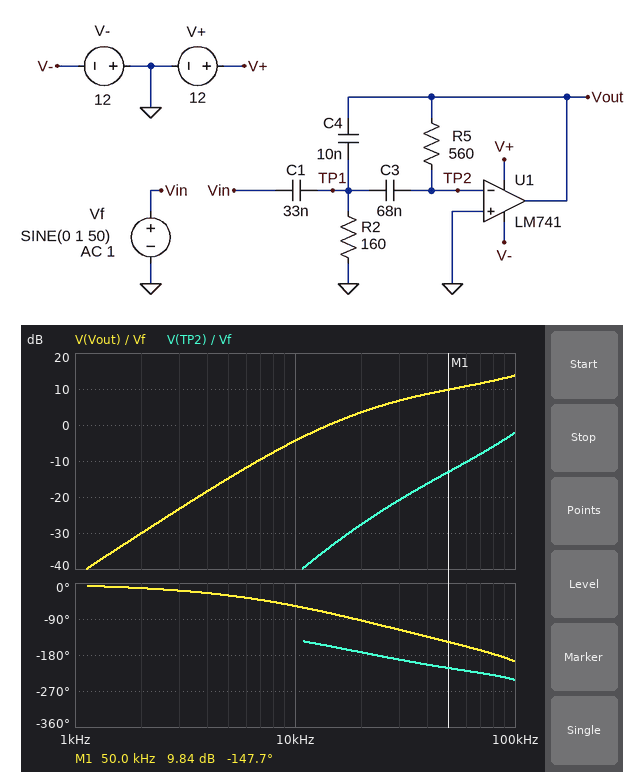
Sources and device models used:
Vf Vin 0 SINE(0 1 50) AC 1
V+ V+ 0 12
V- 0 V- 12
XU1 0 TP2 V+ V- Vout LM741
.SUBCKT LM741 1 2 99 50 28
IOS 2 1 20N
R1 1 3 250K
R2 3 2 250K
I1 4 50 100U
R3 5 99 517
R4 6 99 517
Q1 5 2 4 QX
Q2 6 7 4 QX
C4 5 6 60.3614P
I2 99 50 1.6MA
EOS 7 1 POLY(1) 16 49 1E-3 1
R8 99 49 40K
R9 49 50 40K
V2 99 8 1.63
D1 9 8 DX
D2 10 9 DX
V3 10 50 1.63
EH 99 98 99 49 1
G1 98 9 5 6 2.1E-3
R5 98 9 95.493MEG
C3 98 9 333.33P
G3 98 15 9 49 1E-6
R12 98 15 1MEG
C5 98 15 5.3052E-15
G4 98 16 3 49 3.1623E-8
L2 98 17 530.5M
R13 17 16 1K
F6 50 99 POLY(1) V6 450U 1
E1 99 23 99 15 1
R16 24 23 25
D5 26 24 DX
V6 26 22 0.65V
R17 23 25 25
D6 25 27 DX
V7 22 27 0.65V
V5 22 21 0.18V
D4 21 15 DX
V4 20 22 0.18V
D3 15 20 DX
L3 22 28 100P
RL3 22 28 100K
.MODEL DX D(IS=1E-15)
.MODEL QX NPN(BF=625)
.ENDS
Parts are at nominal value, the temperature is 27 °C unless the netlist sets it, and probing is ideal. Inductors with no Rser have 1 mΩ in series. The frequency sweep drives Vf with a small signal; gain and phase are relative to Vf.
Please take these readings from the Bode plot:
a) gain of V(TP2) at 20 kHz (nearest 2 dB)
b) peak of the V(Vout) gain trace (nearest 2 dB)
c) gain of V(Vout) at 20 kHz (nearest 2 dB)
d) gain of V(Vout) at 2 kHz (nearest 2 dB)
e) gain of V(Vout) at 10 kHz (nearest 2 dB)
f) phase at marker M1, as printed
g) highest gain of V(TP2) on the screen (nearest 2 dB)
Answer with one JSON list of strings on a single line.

["-28 dB", "14 dB", "4 dB", "-30 dB", "-4 dB", "-147.7 deg", "-2 dB"]
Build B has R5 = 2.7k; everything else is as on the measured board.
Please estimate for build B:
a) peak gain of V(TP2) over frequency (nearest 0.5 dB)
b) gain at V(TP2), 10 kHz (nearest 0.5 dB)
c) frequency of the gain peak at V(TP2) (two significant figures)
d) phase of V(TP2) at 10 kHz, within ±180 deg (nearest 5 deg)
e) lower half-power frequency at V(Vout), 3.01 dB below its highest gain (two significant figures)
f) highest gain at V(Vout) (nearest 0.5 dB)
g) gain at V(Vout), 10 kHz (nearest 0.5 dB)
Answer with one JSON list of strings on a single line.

["4.0 dB", "-28.5 dB", "190 kHz", "170 deg", "77 kHz", "14.5 dB", "11.0 dB"]
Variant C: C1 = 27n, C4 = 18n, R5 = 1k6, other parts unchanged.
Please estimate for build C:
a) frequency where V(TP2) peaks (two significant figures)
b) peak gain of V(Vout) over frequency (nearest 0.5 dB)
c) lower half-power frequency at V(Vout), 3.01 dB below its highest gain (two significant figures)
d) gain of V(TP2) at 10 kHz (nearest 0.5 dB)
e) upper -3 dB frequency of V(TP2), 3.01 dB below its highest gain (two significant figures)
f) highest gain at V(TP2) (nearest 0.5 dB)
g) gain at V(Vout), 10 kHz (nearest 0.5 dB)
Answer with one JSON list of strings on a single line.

["200 kHz", "13.0 dB", "130 kHz", "-34.5 dB", "310 kHz", "6.0 dB", "4.0 dB"]
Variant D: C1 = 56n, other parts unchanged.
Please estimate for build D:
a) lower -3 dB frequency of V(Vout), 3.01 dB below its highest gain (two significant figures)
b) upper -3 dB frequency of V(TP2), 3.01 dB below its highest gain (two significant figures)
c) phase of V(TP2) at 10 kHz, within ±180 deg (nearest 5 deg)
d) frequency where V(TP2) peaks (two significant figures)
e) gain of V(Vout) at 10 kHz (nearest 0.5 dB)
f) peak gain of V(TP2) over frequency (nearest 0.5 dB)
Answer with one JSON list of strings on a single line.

["67 kHz", "220 kHz", "-145 deg", "120 kHz", "-1.0 dB", "5.5 dB"]
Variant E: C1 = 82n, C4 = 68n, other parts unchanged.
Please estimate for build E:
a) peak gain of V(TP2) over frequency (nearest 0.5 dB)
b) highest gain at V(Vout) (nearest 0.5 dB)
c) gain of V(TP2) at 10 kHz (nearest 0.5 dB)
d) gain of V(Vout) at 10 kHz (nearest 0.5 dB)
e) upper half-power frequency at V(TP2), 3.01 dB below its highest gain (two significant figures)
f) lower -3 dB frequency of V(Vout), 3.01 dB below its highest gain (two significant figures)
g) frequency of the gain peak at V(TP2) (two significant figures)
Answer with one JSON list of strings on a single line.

["12.5 dB", "19.0 dB", "-36.0 dB", "-1.0 dB", "120 kHz", "90 kHz", "100 kHz"]
